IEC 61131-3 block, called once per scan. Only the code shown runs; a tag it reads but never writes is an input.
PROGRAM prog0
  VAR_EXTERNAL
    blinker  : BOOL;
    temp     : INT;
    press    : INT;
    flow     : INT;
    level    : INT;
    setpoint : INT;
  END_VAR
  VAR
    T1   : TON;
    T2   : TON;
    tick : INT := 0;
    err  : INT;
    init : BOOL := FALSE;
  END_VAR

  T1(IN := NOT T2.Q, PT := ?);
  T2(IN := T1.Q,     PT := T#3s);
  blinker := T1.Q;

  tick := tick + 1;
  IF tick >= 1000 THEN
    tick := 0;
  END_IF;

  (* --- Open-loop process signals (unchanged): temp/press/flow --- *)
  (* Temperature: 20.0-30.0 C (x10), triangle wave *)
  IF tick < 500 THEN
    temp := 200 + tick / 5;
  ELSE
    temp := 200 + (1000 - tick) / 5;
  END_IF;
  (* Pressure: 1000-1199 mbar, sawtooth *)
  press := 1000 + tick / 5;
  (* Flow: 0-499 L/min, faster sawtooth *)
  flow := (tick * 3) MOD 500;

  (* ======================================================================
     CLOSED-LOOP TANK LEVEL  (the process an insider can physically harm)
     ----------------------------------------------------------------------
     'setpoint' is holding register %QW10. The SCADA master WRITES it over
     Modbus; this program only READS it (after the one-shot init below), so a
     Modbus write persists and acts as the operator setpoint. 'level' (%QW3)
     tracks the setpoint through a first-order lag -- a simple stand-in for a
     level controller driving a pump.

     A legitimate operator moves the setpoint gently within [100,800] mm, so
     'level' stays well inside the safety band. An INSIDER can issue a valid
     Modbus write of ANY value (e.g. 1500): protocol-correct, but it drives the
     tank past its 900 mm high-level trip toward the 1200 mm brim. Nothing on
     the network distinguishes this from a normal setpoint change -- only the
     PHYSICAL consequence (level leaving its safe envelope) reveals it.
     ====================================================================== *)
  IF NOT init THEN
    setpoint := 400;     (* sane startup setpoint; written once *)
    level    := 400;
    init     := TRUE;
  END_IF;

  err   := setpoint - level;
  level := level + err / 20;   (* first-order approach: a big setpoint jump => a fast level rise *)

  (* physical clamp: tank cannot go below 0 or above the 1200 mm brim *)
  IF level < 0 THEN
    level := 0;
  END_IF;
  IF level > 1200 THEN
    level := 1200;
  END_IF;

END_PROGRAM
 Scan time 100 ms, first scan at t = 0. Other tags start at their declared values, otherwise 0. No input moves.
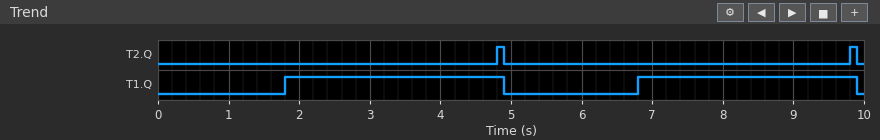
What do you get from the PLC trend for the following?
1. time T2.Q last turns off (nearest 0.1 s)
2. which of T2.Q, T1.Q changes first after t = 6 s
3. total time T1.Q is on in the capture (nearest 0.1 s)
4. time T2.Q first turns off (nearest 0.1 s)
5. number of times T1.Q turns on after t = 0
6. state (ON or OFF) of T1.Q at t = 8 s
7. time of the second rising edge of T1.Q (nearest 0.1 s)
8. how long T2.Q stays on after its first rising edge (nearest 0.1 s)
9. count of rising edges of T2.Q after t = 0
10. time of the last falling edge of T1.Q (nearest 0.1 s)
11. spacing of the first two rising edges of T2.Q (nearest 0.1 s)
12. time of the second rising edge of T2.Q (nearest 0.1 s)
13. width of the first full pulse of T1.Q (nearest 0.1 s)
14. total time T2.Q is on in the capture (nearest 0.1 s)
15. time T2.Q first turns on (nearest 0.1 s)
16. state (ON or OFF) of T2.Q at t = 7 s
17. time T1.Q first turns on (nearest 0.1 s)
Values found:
9.9 s
T1.Q
6.2 s
4.9 s
2
ON
6.8 s
0.1 s
2
9.9 s
5.0 s
9.8 s
3.1 s
0.2 s
4.8 s
OFF
1.8 s
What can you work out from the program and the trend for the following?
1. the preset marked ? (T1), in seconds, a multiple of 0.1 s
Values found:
1.8 s
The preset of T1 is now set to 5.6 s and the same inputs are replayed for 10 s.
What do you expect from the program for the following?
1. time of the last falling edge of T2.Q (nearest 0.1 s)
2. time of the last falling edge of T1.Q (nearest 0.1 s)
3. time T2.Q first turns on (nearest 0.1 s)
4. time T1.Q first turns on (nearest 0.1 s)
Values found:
8.7 s
8.7 s
8.6 s
5.6 s
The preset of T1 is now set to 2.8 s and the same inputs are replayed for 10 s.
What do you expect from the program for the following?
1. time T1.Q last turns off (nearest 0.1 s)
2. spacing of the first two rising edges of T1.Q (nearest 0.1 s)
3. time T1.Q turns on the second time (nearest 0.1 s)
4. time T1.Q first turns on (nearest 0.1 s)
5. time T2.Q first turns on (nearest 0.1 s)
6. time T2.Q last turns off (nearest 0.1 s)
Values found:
5.9 s
6.0 s
8.8 s
2.8 s
5.8 s
5.9 s
